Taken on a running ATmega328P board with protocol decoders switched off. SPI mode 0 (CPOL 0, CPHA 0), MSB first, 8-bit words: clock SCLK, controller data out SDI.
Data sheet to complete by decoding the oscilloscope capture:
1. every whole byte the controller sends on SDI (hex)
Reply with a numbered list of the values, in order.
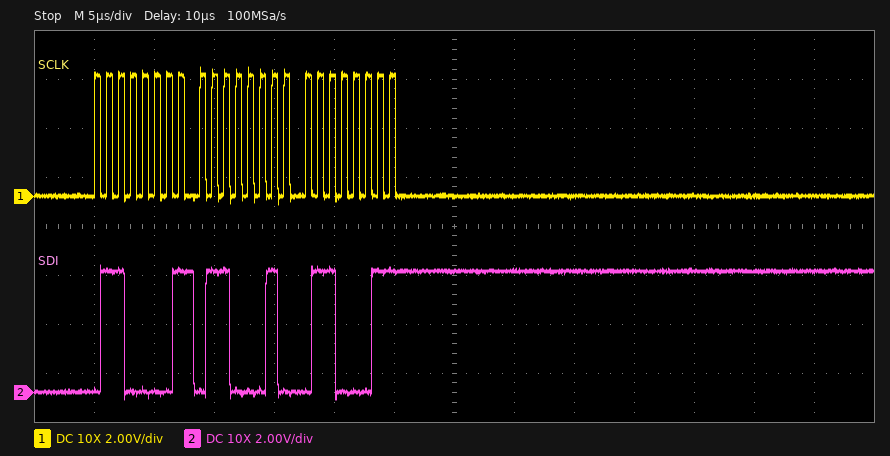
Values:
1. 61 62 63
